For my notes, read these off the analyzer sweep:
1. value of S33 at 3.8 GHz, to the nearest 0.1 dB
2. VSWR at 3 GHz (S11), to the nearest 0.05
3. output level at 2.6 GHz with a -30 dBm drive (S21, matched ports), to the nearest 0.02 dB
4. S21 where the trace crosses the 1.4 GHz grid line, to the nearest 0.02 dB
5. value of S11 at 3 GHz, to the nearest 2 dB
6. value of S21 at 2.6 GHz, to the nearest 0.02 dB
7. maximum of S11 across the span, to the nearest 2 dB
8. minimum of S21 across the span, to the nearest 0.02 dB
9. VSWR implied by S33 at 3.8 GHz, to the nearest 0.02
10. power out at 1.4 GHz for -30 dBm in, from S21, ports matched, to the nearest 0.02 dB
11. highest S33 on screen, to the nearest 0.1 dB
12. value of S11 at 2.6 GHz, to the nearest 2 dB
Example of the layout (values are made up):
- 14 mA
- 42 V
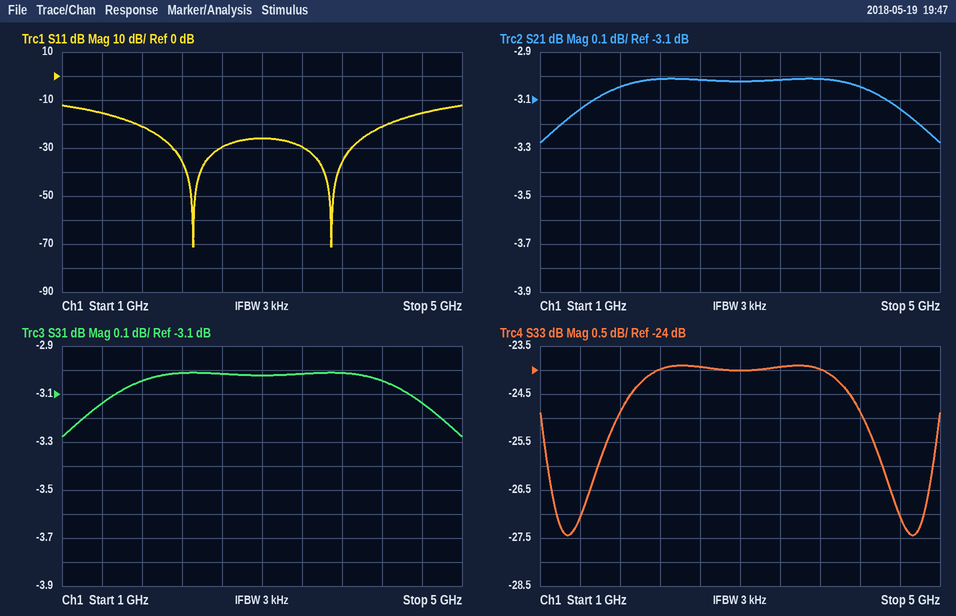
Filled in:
- -24.0 dB
- 1.10
- -33.02 dBm
- -3.14 dB
- -26 dB
- -3.02 dB
- -12 dB
- -3.28 dB
- 1.14
- -33.14 dBm
- -23.9 dB
- -30 dB
